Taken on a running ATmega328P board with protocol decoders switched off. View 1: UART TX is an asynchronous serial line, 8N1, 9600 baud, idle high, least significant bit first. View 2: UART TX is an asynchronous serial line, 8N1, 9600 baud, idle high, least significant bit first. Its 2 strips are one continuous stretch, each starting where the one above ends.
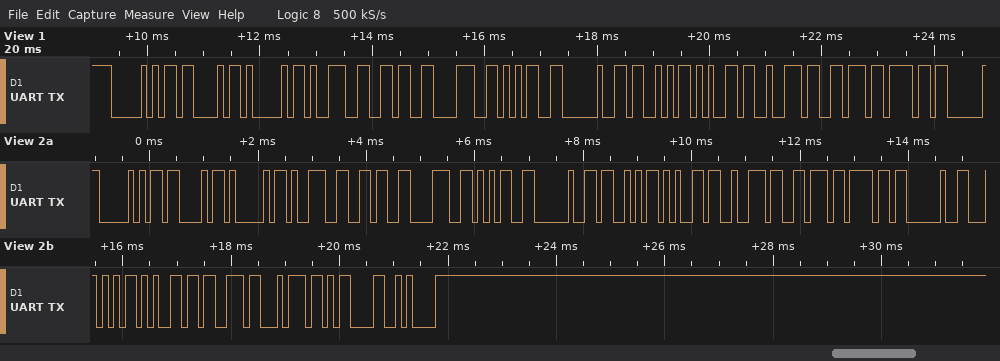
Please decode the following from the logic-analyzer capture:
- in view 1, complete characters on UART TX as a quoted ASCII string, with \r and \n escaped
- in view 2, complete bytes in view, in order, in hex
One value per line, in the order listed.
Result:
"PCA9685 Servo"
50 43 41 39 36 38 35 20 53 65 72 76 6F 20 54 65 73 74 0D 0A
